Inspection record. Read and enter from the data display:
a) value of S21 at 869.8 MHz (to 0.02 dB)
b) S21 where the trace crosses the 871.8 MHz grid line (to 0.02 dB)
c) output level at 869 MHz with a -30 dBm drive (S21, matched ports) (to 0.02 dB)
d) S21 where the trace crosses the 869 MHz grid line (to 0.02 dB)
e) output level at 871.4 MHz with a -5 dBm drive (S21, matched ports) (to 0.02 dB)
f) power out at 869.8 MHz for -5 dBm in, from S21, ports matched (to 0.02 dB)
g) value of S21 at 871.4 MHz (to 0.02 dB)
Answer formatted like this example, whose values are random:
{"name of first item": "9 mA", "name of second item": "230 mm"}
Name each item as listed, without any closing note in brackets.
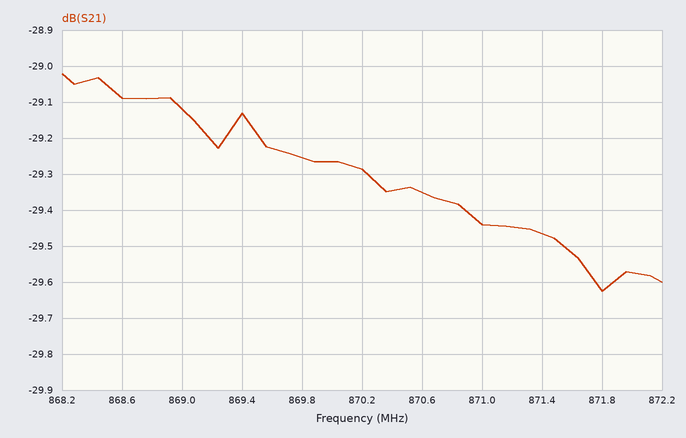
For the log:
{"value of S21 at 869.8 MHz": "-29.26 dB", "S21 where the trace crosses the 871.8 MHz grid line": "-29.62 dB", "output level at 869 MHz with a -30 dBm drive (S21, matched ports)": "-59.12 dBm", "S21 where the trace crosses the 869 MHz grid line": "-29.12 dB", "output level at 871.4 MHz with a -5 dBm drive (S21, matched ports)": "-34.46 dBm", "power out at 869.8 MHz for -5 dBm in, from S21, ports matched": "-34.26 dBm", "value of S21 at 871.4 MHz": "-29.46 dB"}
